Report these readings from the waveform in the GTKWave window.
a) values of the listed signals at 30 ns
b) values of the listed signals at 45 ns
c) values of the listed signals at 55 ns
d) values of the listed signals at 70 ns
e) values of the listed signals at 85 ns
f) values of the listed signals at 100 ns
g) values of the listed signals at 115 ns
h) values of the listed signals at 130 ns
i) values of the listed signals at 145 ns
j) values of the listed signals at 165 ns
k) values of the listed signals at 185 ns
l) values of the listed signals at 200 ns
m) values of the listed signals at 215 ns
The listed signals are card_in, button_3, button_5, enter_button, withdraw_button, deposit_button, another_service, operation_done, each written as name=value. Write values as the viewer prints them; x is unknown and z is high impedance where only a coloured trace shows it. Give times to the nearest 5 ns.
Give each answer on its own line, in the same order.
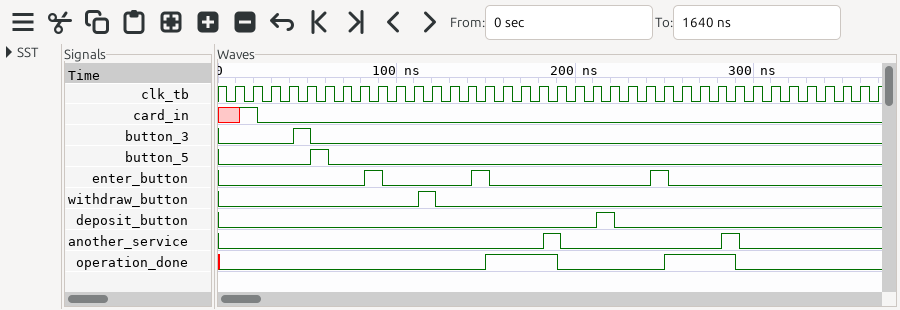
card_in=0, button_3=0, button_5=0, enter_button=0, withdraw_button=0, deposit_button=0, another_service=0, operation_done=0
card_in=0, button_3=1, button_5=0, enter_button=0, withdraw_button=0, deposit_button=0, another_service=0, operation_done=0
card_in=0, button_3=0, button_5=1, enter_button=0, withdraw_button=0, deposit_button=0, another_service=0, operation_done=0
card_in=0, button_3=0, button_5=0, enter_button=0, withdraw_button=0, deposit_button=0, another_service=0, operation_done=0
card_in=0, button_3=0, button_5=0, enter_button=1, withdraw_button=0, deposit_button=0, another_service=0, operation_done=0
card_in=0, button_3=0, button_5=0, enter_button=0, withdraw_button=0, deposit_button=0, another_service=0, operation_done=0
card_in=0, button_3=0, button_5=0, enter_button=0, withdraw_button=1, deposit_button=0, another_service=0, operation_done=0
card_in=0, button_3=0, button_5=0, enter_button=0, withdraw_button=0, deposit_button=0, another_service=0, operation_done=0
card_in=0, button_3=0, button_5=0, enter_button=1, withdraw_button=0, deposit_button=0, another_service=0, operation_done=0
card_in=0, button_3=0, button_5=0, enter_button=0, withdraw_button=0, deposit_button=0, another_service=0, operation_done=1
card_in=0, button_3=0, button_5=0, enter_button=0, withdraw_button=0, deposit_button=0, another_service=1, operation_done=1
card_in=0, button_3=0, button_5=0, enter_button=0, withdraw_button=0, deposit_button=0, another_service=0, operation_done=0
card_in=0, button_3=0, button_5=0, enter_button=0, withdraw_button=0, deposit_button=1, another_service=0, operation_done=0
